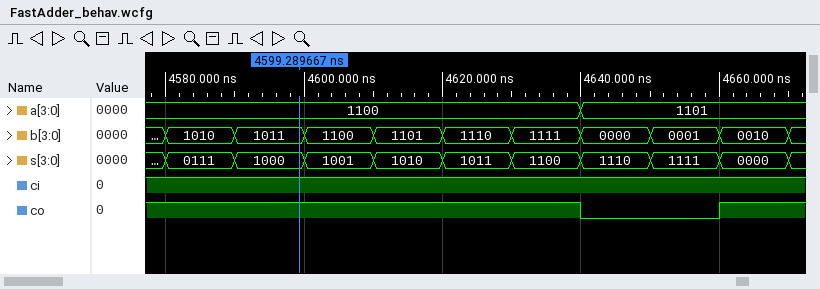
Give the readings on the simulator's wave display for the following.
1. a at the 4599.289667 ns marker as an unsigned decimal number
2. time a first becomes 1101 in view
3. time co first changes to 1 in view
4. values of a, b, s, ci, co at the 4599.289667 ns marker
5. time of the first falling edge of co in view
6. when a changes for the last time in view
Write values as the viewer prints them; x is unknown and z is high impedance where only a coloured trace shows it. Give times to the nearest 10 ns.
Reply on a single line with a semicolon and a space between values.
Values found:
12; 4640 ns; 4660 ns; a=1100, b=1011, s=1000, ci=1, co=1; 4640 ns; 4640 ns
